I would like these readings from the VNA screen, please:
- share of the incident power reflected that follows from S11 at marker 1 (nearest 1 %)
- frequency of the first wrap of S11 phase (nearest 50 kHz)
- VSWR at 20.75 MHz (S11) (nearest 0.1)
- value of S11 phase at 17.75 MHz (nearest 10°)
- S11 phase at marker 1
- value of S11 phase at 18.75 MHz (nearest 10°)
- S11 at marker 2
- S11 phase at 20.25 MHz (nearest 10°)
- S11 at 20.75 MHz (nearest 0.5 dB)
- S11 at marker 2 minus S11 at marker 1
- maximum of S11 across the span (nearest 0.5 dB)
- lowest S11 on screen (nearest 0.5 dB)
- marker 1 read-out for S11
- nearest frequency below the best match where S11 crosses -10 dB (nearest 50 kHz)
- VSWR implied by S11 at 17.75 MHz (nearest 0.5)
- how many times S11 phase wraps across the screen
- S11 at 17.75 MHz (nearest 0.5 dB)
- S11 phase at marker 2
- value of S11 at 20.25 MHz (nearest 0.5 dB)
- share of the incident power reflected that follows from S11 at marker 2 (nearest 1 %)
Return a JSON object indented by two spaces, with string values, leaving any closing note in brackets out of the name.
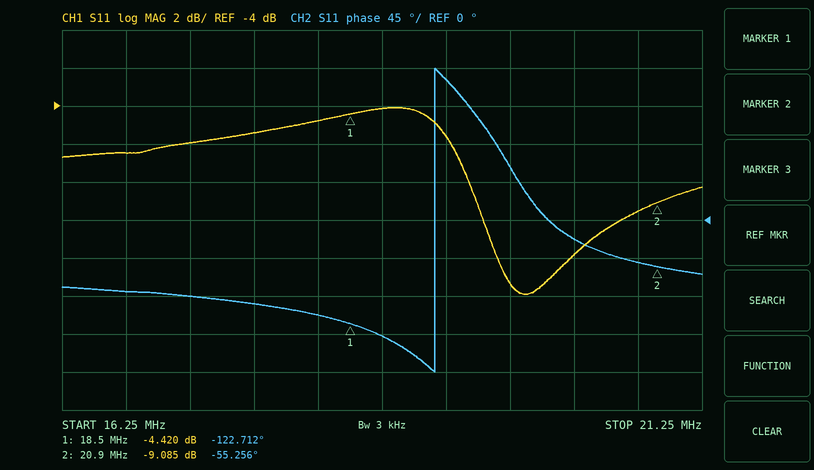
{
  "share of the incident power reflected that follows from S11 at marker 1": "36 %",
  "frequency of the first wrap of S11 phase": "19.15 MHz",
  "VSWR at 20.75 MHz (S11)": "2.0",
  "value of S11 phase at 17.75 MHz": "-100°",
  "S11 phase at marker 1": "-122.712°",
  "value of S11 phase at 18.75 MHz": "-140°",
  "S11 at marker 2": "-9.085 dB",
  "S11 phase at 20.25 MHz": "-20°",
  "S11 at 20.75 MHz": "-9.5 dB",
  "S11 at marker 2 minus S11 at marker 1": "-4.665 dB",
  "maximum of S11 across the span": "-4.0 dB",
  "lowest S11 on screen": "-14.0 dB",
  "marker 1 read-out for S11": "-4.420 dB",
  "nearest frequency below the best match where S11 crosses -10 dB": "19.55 MHz",
  "VSWR implied by S11 at 17.75 MHz": "3.5",
  "how many times S11 phase wraps across the screen": "1",
  "S11 at 17.75 MHz": "-5.5 dB",
  "S11 phase at marker 2": "-55.256°",
  "value of S11 at 20.25 MHz": "-12.0 dB",
  "share of the incident power reflected that follows from S11 at marker 2": "12 %"
}
